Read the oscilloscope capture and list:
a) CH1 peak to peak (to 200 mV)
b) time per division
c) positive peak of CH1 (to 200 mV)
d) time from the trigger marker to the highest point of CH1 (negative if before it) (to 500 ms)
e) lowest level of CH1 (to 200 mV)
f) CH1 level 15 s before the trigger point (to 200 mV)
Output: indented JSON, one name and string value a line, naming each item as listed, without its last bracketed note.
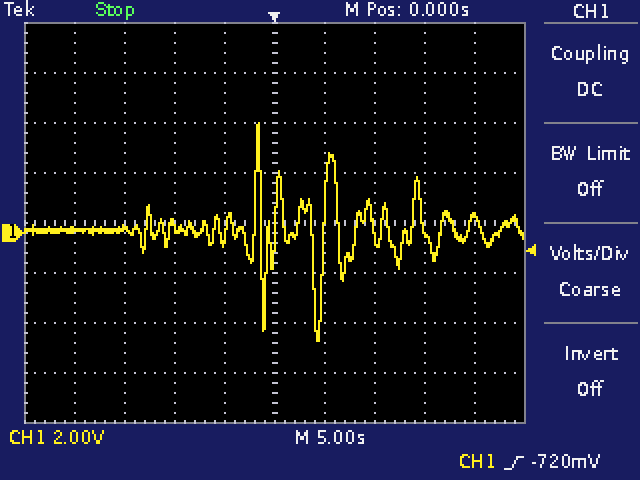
{
  "CH1 peak to peak": "8.8 V",
  "time per division": "5 s",
  "positive peak of CH1": "4.4 V",
  "time from the trigger marker to the highest point of CH1 (negative if before it)": "-1.5 s",
  "lowest level of CH1": "-4.4 V",
  "CH1 level 15 s before the trigger point": "200 mV"
}
